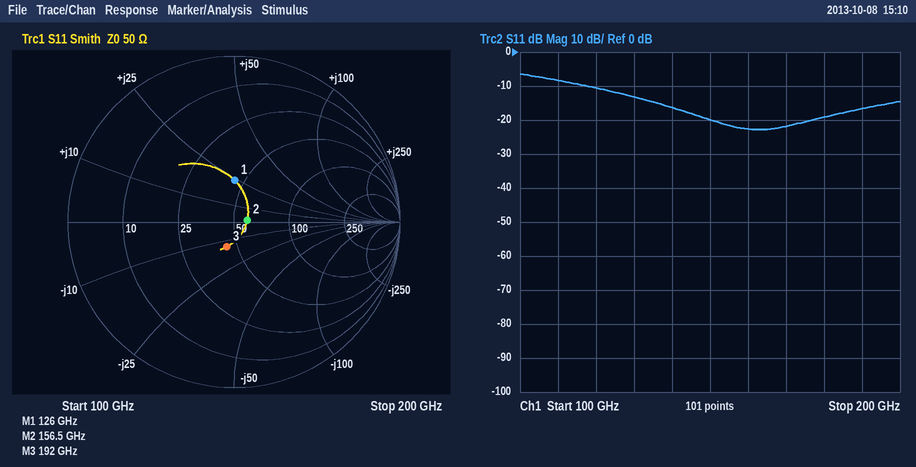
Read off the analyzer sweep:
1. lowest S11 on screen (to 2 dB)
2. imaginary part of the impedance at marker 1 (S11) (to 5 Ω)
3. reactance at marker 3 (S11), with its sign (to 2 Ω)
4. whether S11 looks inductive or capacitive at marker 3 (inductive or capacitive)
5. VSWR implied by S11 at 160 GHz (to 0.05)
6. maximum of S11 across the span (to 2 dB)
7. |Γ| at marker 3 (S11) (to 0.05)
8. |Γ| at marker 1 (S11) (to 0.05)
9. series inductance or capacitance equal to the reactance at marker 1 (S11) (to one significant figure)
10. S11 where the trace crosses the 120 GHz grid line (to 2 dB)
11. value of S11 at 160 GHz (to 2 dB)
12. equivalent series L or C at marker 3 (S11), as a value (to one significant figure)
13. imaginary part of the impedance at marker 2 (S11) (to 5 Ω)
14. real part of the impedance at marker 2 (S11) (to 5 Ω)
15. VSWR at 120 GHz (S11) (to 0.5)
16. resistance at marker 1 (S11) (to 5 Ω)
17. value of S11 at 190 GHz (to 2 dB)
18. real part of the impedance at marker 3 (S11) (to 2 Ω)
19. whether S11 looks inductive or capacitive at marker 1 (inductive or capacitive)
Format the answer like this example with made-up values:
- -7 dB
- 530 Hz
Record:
- -22 dB
- +25 Ω
- -14 Ω
- capacitive
- 1.15
- -6 dB
- 0.15
- 0.25
- 30 pH
- -10 dB
- -22 dB
- 60 fF
- 0 Ω
- 60 Ω
- 2.0
- 45 Ω
- -16 dB
- 44 Ω
- inductive
